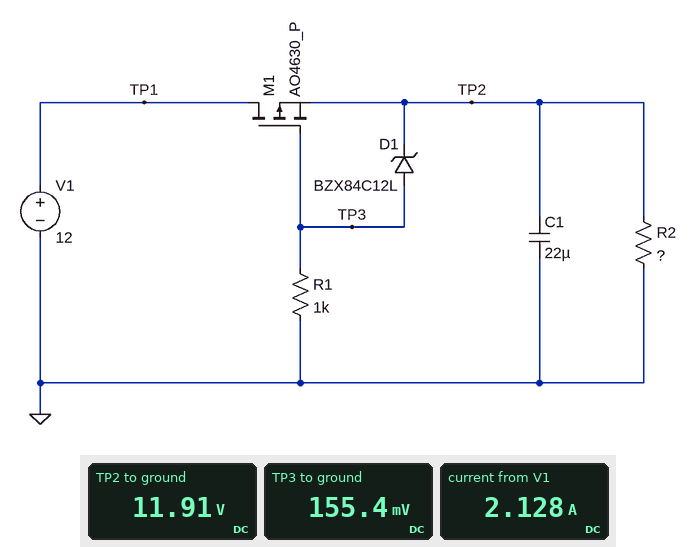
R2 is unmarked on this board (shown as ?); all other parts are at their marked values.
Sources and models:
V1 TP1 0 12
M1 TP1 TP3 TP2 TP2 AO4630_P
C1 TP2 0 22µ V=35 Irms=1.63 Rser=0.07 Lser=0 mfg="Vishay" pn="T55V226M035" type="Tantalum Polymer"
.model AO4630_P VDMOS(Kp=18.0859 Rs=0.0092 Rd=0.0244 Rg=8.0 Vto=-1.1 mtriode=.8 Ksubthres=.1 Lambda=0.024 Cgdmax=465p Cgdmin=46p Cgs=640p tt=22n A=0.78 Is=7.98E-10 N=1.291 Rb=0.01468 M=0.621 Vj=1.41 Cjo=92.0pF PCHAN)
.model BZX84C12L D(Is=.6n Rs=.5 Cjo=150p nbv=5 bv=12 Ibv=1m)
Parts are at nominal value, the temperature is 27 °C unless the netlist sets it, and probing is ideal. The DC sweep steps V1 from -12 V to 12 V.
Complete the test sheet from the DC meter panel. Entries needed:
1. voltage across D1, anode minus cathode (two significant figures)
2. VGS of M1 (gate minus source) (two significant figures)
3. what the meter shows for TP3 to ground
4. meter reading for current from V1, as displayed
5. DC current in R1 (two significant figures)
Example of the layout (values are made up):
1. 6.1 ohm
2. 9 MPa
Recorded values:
1. -12 V
2. -12 V
3. 155.4 mV
4. 2.128 A
5. 160 µA
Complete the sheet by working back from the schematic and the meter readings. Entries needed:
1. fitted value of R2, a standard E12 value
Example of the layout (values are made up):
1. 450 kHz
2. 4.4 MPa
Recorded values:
1. 5.6 Ω
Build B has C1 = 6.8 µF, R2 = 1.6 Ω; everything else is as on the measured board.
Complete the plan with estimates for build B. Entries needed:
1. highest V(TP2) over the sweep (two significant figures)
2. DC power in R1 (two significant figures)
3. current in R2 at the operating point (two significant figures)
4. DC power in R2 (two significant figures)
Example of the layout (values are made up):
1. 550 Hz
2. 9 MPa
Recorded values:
1. 12 V
2. 4.0 µW
3. 7.3 A
4. 86 W
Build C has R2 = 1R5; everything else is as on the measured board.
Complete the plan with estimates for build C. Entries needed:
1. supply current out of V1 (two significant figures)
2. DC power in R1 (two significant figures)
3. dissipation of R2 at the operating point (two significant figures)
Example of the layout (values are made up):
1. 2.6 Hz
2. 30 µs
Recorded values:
1. 7.8 A
2. 3.3 µW
3. 91 W
